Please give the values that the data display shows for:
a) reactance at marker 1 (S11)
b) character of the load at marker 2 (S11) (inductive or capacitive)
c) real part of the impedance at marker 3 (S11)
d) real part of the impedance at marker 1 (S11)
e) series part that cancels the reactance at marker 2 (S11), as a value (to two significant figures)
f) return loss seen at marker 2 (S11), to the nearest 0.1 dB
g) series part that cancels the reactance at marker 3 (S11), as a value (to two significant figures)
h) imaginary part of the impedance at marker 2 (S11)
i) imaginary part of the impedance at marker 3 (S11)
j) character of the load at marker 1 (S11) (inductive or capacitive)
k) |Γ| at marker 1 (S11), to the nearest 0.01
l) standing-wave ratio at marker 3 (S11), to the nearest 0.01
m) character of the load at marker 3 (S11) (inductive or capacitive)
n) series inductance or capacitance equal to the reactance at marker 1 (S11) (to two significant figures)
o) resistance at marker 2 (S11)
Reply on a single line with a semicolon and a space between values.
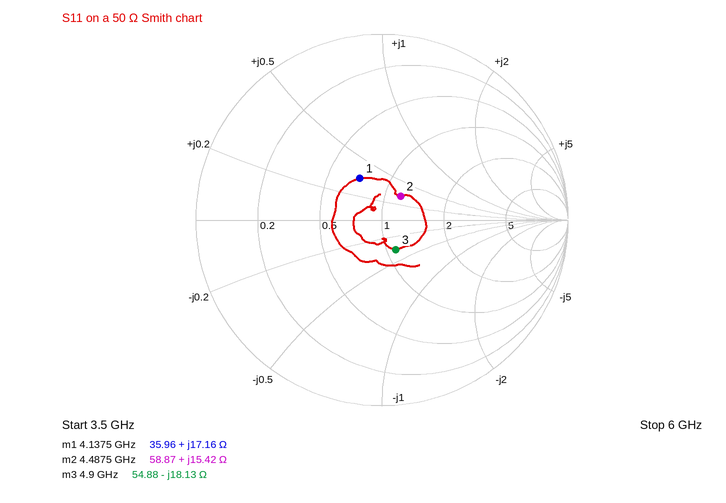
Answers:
+17.16 Ω; inductive; 54.88 Ω; 35.96 Ω; 2.3 pF; 15.8 dB; 590 pH; +15.42 Ω; -18.13 Ω; inductive; 0.25; 1.43; capacitive; 660 pH; 58.87 Ω
